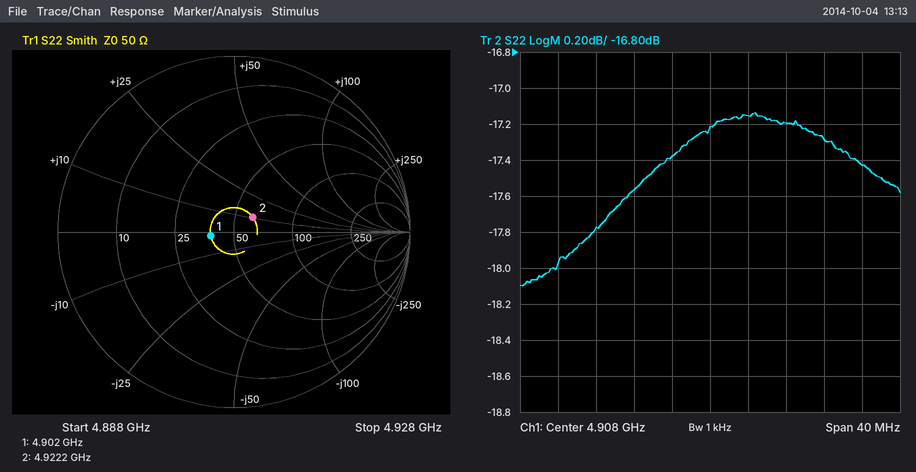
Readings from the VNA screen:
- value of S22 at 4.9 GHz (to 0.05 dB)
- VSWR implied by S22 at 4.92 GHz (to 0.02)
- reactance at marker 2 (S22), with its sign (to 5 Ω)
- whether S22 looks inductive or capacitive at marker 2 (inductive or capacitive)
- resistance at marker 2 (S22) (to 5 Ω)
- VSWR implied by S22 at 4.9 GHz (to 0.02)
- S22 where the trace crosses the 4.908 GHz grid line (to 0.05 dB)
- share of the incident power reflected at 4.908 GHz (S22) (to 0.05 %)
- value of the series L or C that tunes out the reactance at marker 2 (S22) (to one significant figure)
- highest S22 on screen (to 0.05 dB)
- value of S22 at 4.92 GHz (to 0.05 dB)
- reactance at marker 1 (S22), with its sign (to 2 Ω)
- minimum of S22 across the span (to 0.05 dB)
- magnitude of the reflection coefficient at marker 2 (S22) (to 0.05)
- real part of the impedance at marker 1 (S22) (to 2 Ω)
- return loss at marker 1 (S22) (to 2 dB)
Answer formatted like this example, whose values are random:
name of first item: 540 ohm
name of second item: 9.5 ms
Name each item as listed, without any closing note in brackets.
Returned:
value of S22 at 4.9 GHz: -17.55 dB
VSWR implied by S22 at 4.92 GHz: 1.32
reactance at marker 2 (S22), with its sign: +10 Ω
whether S22 looks inductive or capacitive at marker 2: inductive
resistance at marker 2 (S22): 60 Ω
VSWR implied by S22 at 4.9 GHz: 1.30
S22 where the trace crosses the 4.908 GHz grid line: -17.20 dB
share of the incident power reflected at 4.908 GHz (S22): 1.90 %
value of the series L or C that tunes out the reactance at marker 2 (S22): 3 pF
highest S22 on screen: -17.15 dB
value of S22 at 4.92 GHz: -17.30 dB
reactance at marker 1 (S22), with its sign: -2 Ω
minimum of S22 across the span: -18.10 dB
magnitude of the reflection coefficient at marker 2 (S22): 0.15
real part of the impedance at marker 1 (S22): 38 Ω
return loss at marker 1 (S22): 18 dB
